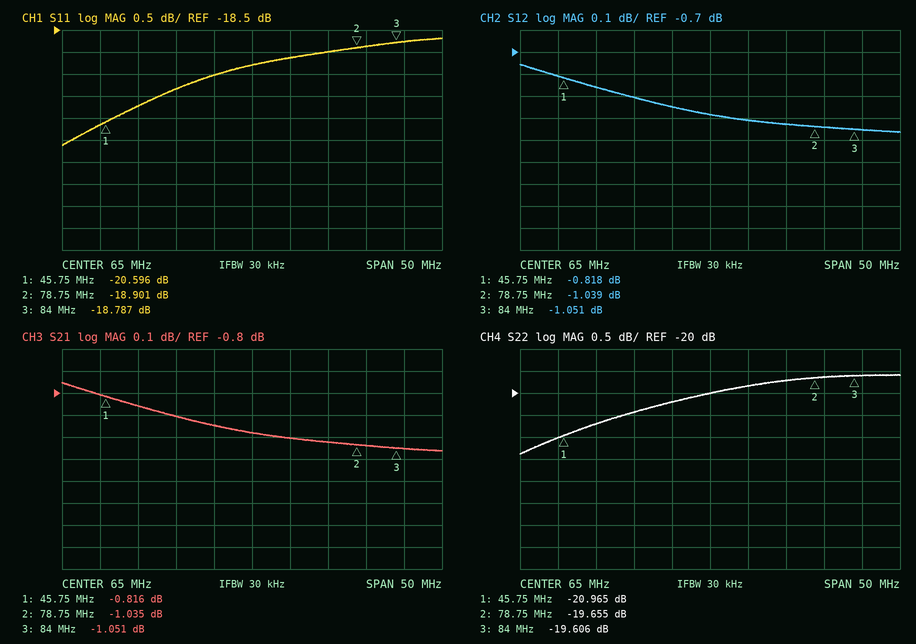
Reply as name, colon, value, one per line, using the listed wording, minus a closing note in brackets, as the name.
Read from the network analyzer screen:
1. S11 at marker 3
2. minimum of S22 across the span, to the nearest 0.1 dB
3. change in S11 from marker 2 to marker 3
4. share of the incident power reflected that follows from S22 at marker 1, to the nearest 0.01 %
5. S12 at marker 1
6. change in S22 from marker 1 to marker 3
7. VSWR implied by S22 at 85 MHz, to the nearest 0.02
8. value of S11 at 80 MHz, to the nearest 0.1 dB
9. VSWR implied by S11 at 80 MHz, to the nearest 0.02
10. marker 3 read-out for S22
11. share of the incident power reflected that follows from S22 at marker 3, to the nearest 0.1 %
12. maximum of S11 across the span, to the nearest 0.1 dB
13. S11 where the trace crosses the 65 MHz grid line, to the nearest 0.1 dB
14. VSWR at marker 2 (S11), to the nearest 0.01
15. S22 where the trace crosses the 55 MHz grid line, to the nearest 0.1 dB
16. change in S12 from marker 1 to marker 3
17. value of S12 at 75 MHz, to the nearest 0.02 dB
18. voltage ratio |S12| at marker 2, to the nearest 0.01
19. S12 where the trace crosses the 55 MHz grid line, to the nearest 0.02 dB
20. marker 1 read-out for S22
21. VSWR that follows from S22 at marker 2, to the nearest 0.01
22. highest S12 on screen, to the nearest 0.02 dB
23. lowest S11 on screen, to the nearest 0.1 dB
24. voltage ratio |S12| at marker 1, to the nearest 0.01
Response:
S11 at marker 3: -18.787 dB
minimum of S22 across the span, to the nearest 0.1 dB: -21.4 dB
change in S11 from marker 2 to marker 3: 0.114 dB
share of the incident power reflected that follows from S22 at marker 1, to the nearest 0.01 %: 0.80 %
S12 at marker 1: -0.818 dB
change in S22 from marker 1 to marker 3: 1.359 dB
VSWR implied by S22 at 85 MHz, to the nearest 0.02: 1.24
value of S11 at 80 MHz, to the nearest 0.1 dB: -18.9 dB
VSWR implied by S11 at 80 MHz, to the nearest 0.02: 1.26
marker 3 read-out for S22: -19.606 dB
share of the incident power reflected that follows from S22 at marker 3, to the nearest 0.1 %: 1.1 %
maximum of S11 across the span, to the nearest 0.1 dB: -18.7 dB
S11 where the trace crosses the 65 MHz grid line, to the nearest 0.1 dB: -19.3 dB
VSWR at marker 2 (S11), to the nearest 0.01: 1.26
S22 where the trace crosses the 55 MHz grid line, to the nearest 0.1 dB: -20.4 dB
change in S12 from marker 1 to marker 3: -0.233 dB
value of S12 at 75 MHz, to the nearest 0.02 dB: -1.02 dB
voltage ratio |S12| at marker 2, to the nearest 0.01: 0.89
S12 where the trace crosses the 55 MHz grid line, to the nearest 0.02 dB: -0.90 dB
marker 1 read-out for S22: -20.965 dB
VSWR that follows from S22 at marker 2, to the nearest 0.01: 1.23
highest S12 on screen, to the nearest 0.02 dB: -0.76 dB
lowest S11 on screen, to the nearest 0.1 dB: -21.1 dB
voltage ratio |S12| at marker 1, to the nearest 0.01: 0.91
